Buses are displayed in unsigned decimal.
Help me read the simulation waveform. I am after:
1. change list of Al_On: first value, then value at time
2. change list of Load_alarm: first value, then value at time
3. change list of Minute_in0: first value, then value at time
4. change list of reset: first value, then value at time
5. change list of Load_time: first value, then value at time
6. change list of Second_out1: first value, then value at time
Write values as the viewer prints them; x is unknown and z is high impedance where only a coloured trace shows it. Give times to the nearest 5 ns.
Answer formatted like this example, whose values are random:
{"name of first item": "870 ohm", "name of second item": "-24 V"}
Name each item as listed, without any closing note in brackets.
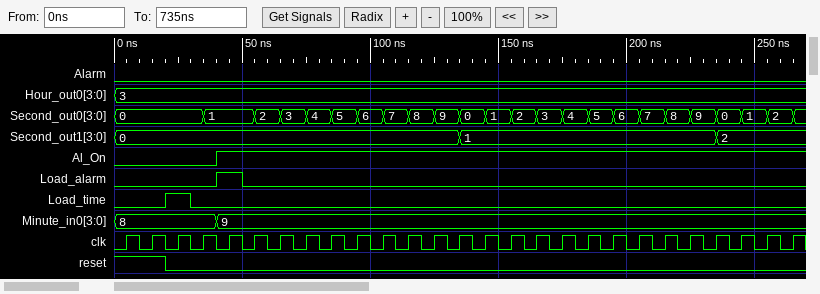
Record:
{"change list of Al_On: first value, then value at time": "0, 1 at 40 ns", "change list of Load_alarm: first value, then value at time": "0, 1 at 40 ns, 0 at 50 ns", "change list of Minute_in0: first value, then value at time": "8, 9 at 40 ns", "change list of reset: first value, then value at time": "1, 0 at 20 ns", "change list of Load_time: first value, then value at time": "0, 1 at 20 ns, 0 at 30 ns", "change list of Second_out1: first value, then value at time": "0, 1 at 135 ns, 2 at 235 ns"}
